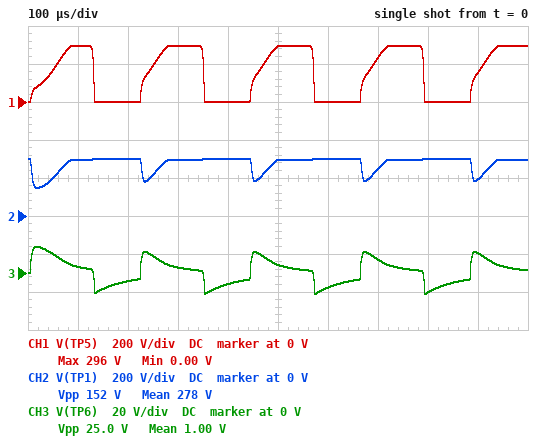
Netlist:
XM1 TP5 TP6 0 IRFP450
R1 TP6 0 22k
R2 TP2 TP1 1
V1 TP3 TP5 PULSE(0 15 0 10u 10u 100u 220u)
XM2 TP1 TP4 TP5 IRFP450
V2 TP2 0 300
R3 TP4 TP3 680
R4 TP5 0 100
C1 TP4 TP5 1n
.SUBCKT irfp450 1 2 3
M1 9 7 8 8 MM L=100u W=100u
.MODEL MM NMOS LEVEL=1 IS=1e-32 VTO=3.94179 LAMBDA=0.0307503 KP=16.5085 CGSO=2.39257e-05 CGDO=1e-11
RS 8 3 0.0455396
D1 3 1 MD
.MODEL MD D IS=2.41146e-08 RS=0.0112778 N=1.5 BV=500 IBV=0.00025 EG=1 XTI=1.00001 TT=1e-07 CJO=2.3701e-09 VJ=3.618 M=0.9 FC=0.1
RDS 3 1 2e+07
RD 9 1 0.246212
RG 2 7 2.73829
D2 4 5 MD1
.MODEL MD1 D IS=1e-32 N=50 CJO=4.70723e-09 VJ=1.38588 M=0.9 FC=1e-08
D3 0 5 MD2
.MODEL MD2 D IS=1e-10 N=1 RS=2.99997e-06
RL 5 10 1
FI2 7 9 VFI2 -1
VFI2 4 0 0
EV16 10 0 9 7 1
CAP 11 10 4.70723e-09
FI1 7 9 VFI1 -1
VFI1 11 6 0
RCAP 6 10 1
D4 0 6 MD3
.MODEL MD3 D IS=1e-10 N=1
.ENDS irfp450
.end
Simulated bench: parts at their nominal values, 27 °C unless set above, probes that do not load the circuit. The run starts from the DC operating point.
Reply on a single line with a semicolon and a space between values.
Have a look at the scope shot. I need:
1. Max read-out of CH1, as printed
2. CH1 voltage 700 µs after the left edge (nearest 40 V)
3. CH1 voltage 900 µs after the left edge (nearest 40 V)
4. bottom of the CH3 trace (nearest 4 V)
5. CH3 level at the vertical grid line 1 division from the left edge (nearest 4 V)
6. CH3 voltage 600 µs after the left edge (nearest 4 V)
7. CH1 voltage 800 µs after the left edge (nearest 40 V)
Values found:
296 V; 240 V; 160 V; -12 V; 4 V; -8 V; 0 V
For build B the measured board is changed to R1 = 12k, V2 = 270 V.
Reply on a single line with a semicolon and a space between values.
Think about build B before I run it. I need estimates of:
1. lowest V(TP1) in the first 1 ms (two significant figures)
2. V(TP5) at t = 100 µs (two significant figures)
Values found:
140 V; 270 V
